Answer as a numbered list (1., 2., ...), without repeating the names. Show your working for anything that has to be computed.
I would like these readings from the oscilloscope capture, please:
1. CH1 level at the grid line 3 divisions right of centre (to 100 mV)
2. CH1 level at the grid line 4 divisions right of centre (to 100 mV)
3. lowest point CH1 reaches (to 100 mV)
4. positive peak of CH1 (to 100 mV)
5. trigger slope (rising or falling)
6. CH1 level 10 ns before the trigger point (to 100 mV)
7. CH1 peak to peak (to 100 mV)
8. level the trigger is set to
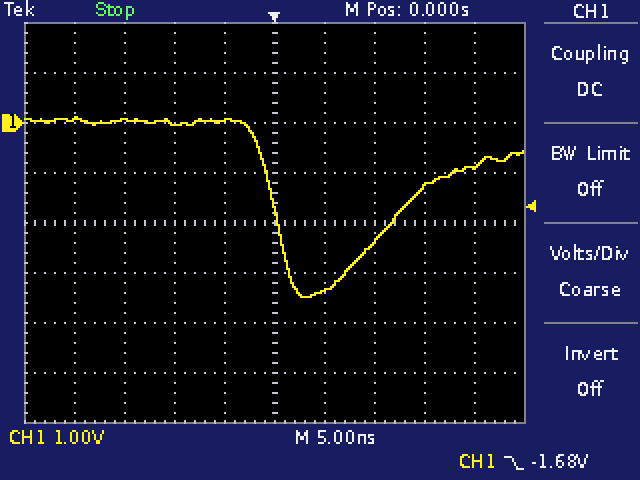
1. -1.3 V
2. -900 mV
3. -3.5 V
4. 100 mV
5. falling
6. 0.0 V
7. 100 mV − (-3.5 V) = 3.6 V
8. -1.68 V
